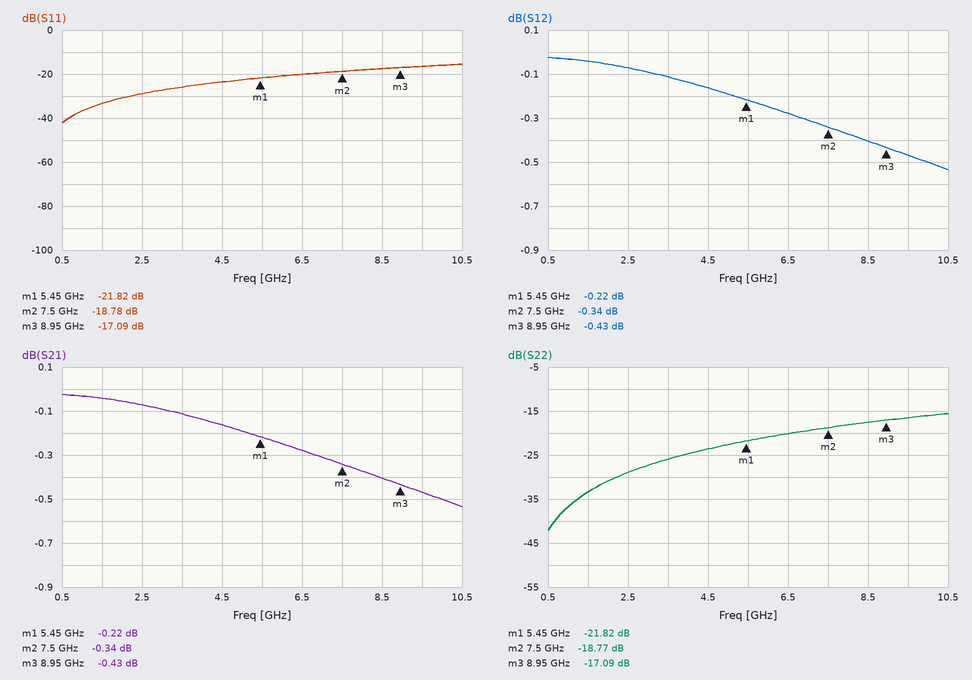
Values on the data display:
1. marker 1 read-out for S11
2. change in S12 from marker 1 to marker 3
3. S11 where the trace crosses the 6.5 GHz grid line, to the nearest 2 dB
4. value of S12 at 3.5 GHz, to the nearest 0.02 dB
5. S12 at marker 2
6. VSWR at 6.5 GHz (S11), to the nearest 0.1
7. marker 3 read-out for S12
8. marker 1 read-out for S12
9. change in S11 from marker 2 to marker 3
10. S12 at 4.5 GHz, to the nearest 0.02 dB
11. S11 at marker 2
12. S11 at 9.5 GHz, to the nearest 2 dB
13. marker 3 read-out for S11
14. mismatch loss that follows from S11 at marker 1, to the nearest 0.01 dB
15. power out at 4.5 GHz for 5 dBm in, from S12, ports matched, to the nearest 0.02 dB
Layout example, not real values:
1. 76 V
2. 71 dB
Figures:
1. -21.82 dB
2. -0.21 dB
3. -20 dB
4. -0.12 dB
5. -0.34 dB
6. 1.2
7. -0.43 dB
8. -0.22 dB
9. 1.69 dB
10. -0.16 dB
11. -18.78 dB
12. -16 dB
13. -17.09 dB
14. 0.03 dB
15. 4.84 dBm
